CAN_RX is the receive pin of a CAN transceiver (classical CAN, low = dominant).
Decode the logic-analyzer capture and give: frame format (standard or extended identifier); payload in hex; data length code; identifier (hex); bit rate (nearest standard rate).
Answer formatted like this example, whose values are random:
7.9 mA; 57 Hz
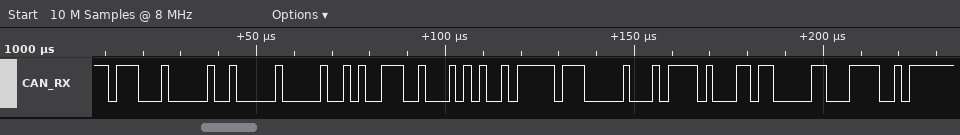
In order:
standard; 00 53 91 52 FF 00 BD 1B; 8; 0x710; 500 kbit/s
